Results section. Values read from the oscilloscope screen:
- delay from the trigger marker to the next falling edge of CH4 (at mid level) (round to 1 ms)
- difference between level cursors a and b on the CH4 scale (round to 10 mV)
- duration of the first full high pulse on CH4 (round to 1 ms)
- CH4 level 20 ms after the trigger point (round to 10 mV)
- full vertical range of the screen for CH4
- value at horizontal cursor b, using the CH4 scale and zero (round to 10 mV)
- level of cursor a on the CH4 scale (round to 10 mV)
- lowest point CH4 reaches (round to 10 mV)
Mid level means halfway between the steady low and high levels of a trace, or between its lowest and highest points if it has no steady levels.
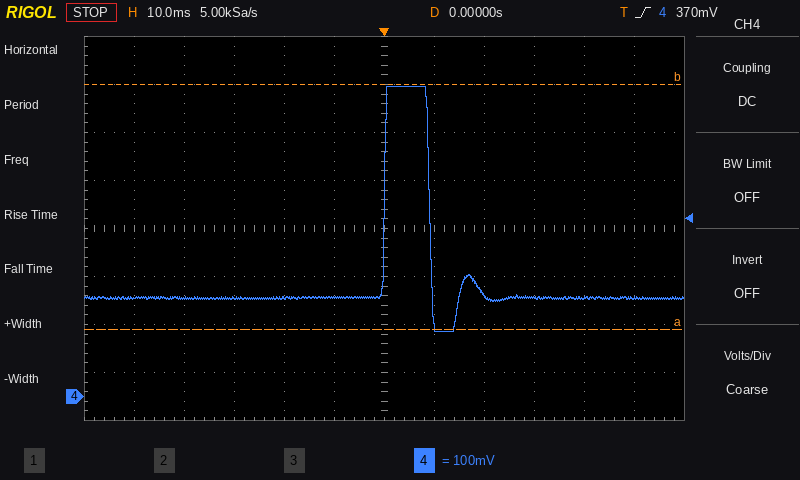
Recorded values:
9 ms
510 mV
9 ms
210 mV
800 mV
650 mV
140 mV
140 mV
